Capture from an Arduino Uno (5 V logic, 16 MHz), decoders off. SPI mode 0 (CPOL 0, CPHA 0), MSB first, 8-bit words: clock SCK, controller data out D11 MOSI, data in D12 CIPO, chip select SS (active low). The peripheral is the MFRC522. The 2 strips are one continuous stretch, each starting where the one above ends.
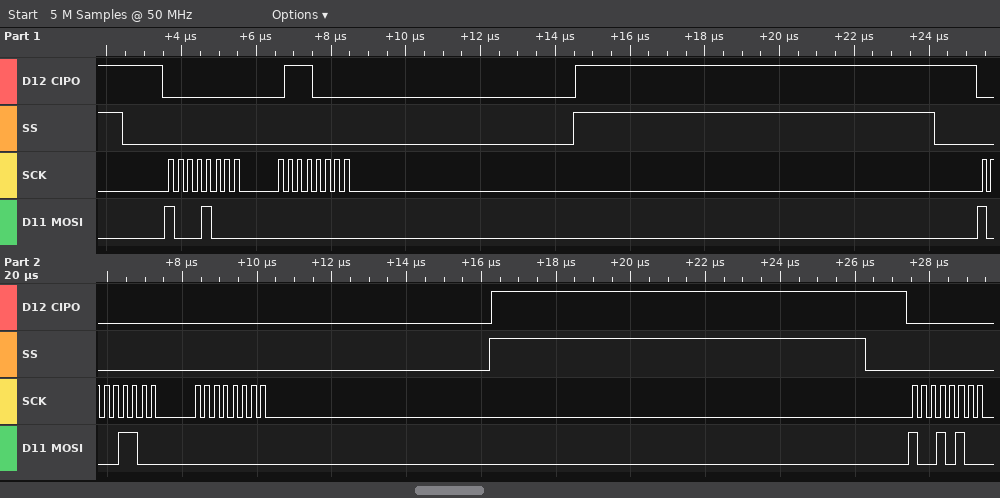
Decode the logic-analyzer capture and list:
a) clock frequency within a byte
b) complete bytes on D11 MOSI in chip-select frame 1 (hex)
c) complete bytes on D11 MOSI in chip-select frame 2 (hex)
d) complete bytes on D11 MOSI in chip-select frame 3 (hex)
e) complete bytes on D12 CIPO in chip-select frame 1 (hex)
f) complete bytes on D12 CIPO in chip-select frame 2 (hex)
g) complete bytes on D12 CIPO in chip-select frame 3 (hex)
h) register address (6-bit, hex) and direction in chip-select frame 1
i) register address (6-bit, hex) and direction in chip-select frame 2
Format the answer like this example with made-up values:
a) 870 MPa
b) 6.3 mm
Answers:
a) 4 MHz
b) 0x88 0x00
c) 0x8C 0x00
d) 0x94
e) 0x00 0x70
f) 0x00 0x00
g) 0x00
h) 0x04 read
i) 0x06 read
